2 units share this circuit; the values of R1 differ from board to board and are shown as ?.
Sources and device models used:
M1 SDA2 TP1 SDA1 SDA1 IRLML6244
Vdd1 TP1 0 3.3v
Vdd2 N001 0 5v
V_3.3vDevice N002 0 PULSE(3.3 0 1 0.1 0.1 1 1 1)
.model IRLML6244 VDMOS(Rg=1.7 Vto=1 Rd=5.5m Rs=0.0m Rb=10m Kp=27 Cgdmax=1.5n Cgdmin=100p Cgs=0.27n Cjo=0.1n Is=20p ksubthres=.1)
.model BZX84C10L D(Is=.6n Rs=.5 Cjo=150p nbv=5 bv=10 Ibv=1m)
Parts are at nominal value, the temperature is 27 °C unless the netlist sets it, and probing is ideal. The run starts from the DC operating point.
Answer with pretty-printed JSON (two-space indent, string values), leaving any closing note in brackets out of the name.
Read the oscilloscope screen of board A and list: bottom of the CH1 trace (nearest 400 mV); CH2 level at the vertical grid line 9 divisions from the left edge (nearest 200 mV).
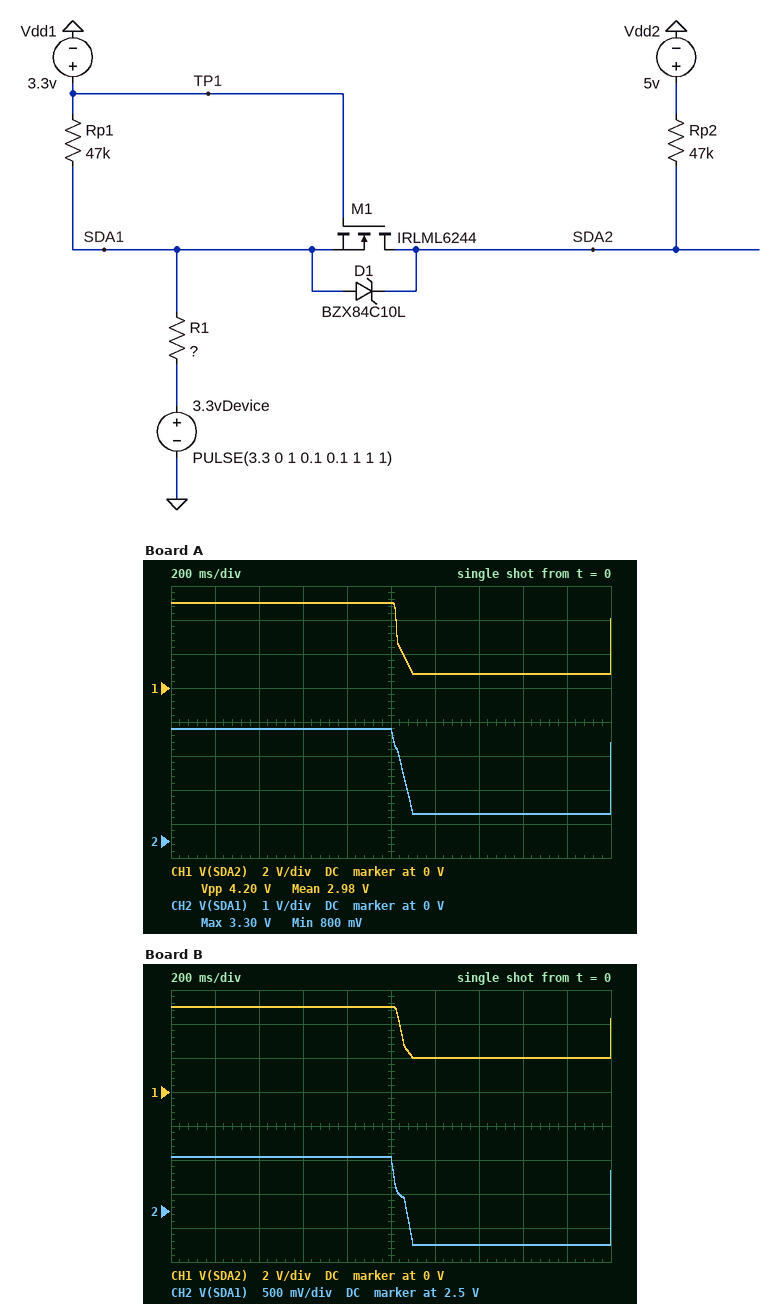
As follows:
{
  "bottom of the CH1 trace": "800 mV",
  "CH2 level at the vertical grid line 9 divisions from the left edge": "800 mV"
}
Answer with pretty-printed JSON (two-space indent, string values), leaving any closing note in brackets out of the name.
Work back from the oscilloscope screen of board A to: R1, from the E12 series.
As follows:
{
  "R1, from the E12 series": "5.6 kΩ"
}
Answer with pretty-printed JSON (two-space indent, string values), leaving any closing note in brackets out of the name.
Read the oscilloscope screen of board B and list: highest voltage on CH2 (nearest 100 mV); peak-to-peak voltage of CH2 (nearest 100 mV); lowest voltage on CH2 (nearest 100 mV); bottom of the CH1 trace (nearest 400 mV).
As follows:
{
  "highest voltage on CH2": "3.3 V",
  "peak-to-peak voltage of CH2": "1.3 V",
  "lowest voltage on CH2": "2.0 V",
  "bottom of the CH1 trace": "2.0 V"
}
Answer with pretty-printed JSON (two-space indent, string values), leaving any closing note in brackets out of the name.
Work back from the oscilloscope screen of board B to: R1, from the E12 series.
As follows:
{
  "R1, from the E12 series": "22 kΩ"
}
